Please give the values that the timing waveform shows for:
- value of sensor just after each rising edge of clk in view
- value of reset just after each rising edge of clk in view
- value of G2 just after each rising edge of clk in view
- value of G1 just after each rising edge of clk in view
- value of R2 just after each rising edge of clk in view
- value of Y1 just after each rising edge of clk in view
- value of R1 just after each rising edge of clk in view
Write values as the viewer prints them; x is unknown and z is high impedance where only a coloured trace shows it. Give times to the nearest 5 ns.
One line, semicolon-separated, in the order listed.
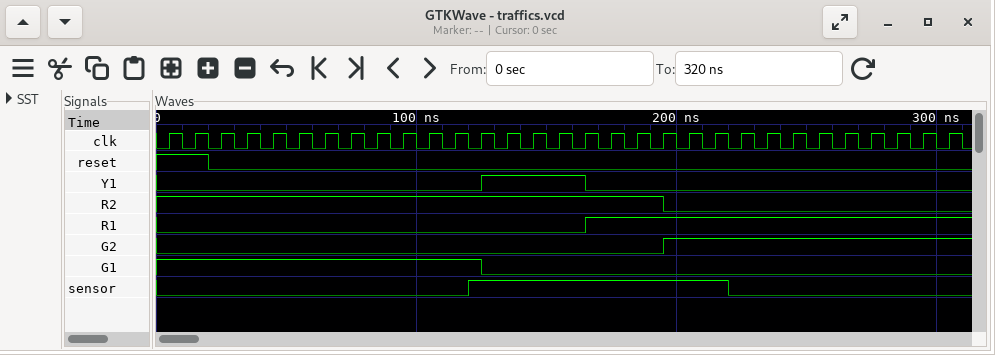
0 0 0 0 0 0 0 0 0 0 0 0 1 1 1 1 1 1 1 1 1 1 0 0 0 0 0 0 0 0 0; 1 1 0 0 0 0 0 0 0 0 0 0 0 0 0 0 0 0 0 0 0 0 0 0 0 0 0 0 0 0 0; 0 0 0 0 0 0 0 0 0 0 0 0 0 0 0 0 0 0 0 1 1 1 1 1 1 1 1 1 1 1 1; 1 1 1 1 1 1 1 1 1 1 1 1 0 0 0 0 0 0 0 0 0 0 0 0 0 0 0 0 0 0 0; 1 1 1 1 1 1 1 1 1 1 1 1 1 1 1 1 1 1 1 0 0 0 0 0 0 0 0 0 0 0 0; 0 0 0 0 0 0 0 0 0 0 0 0 1 1 1 1 0 0 0 0 0 0 0 0 0 0 0 0 0 0 0; 0 0 0 0 0 0 0 0 0 0 0 0 0 0 0 0 1 1 1 1 1 1 1 1 1 1 1 1 1 1 1
